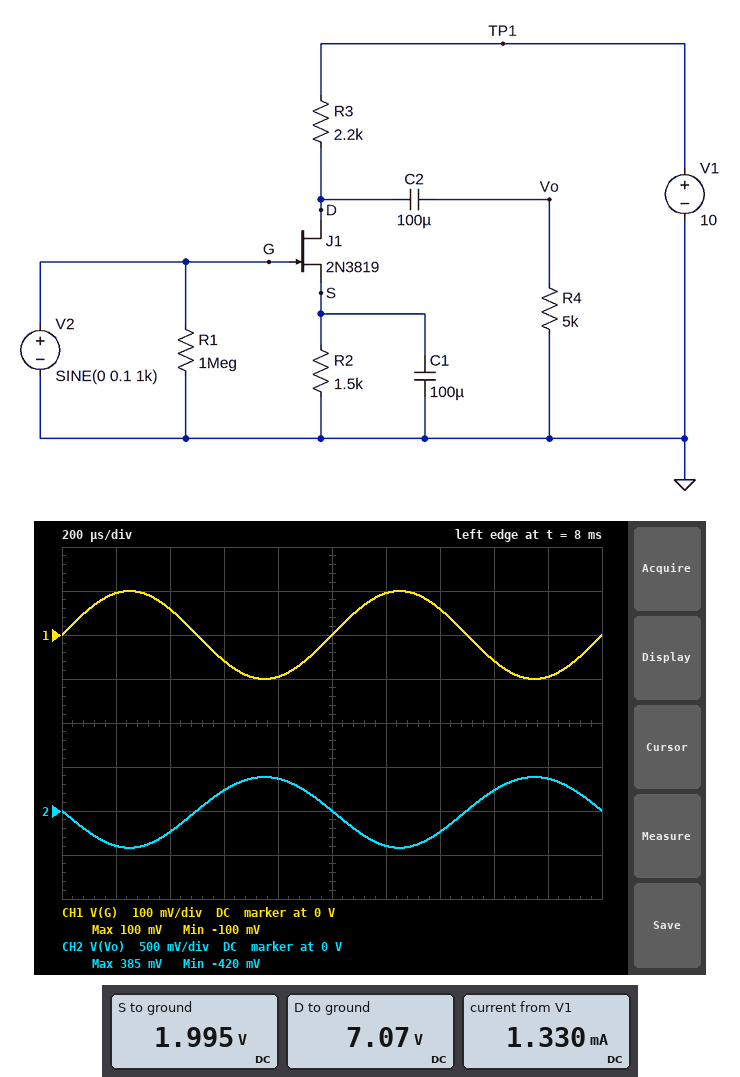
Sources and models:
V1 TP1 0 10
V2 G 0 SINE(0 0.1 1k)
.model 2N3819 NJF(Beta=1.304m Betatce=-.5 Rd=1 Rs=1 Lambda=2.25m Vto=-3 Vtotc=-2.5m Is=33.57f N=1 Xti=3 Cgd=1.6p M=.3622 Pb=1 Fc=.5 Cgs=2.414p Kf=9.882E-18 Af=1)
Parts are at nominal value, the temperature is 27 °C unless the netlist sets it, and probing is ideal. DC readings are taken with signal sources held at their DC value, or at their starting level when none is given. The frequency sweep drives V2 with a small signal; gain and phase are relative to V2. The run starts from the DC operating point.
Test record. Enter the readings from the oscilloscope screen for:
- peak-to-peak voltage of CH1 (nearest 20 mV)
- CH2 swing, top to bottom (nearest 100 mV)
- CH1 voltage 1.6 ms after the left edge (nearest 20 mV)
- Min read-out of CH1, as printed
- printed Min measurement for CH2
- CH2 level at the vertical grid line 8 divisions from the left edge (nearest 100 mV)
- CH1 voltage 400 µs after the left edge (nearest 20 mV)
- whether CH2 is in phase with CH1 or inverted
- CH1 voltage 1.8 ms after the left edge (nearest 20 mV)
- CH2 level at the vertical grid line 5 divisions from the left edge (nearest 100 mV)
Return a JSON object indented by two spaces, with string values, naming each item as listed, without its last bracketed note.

{
  "peak-to-peak voltage of CH1": "200 mV",
  "CH2 swing, top to bottom": "800 mV",
  "CH1 voltage 1.6 ms after the left edge": "-60 mV",
  "Min read-out of CH1, as printed": "-100 mV",
  "printed Min measurement for CH2": "-420 mV",
  "CH2 level at the vertical grid line 8 divisions from the left edge": "200 mV",
  "CH1 voltage 400 µs after the left edge": "60 mV",
  "whether CH2 is in phase with CH1 or inverted": "inverted",
  "CH1 voltage 1.8 ms after the left edge": "-100 mV",
  "CH2 level at the vertical grid line 5 divisions from the left edge": "0 V"
}
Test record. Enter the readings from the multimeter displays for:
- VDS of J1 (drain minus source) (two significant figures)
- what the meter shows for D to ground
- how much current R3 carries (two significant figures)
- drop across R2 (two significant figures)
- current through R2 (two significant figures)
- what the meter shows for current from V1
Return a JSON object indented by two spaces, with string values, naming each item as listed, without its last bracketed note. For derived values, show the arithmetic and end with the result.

{
  "VDS of J1 (drain minus source)": "7.07 V - 1.995 V = 5.1 V",
  "what the meter shows for D to ground": "7.07 V",
  "how much current R3 carries": "(10 V - 7.07 V) / 2.2 kΩ = 1.3 mA",
  "drop across R2": "1.995 V = 2.0 V",
  "current through R2": "(1.995 V) / 1.5 kΩ = 1.3 mA",
  "what the meter shows for current from V1": "1.330 mA"
}
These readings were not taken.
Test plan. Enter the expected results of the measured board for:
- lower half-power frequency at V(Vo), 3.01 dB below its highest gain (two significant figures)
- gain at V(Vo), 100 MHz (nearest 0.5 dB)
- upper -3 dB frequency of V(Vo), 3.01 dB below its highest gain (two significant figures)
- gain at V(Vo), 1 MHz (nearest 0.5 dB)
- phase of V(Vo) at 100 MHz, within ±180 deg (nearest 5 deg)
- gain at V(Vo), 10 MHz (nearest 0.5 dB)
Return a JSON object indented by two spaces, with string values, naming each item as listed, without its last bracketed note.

{
  "lower half-power frequency at V(Vo), 3.01 dB below its highest gain": "5.0 Hz",
  "gain at V(Vo), 100 MHz": "11.0 dB",
  "upper -3 dB frequency of V(Vo), 3.01 dB below its highest gain": "200 MHz",
  "gain at V(Vo), 1 MHz": "12.0 dB",
  "phase of V(Vo) at 100 MHz, within ±180 deg": "145 deg",
  "gain at V(Vo), 10 MHz": "12.0 dB"
}
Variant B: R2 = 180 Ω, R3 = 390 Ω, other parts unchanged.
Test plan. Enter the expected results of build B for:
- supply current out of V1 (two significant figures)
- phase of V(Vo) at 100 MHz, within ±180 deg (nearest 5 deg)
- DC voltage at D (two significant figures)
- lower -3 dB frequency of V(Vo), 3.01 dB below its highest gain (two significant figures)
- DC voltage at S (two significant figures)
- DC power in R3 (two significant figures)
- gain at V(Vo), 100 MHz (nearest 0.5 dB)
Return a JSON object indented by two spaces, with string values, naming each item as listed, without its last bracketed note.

{
  "supply current out of V1": "5.4 mA",
  "phase of V(Vo) at 100 MHz, within ±180 deg": "170 deg",
  "DC voltage at D": "7.9 V",
  "lower -3 dB frequency of V(Vo), 3.01 dB below its highest gain": "12 Hz",
  "DC voltage at S": "970 mV",
  "DC power in R3": "11 mW",
  "gain at V(Vo), 100 MHz": "5.5 dB"
}
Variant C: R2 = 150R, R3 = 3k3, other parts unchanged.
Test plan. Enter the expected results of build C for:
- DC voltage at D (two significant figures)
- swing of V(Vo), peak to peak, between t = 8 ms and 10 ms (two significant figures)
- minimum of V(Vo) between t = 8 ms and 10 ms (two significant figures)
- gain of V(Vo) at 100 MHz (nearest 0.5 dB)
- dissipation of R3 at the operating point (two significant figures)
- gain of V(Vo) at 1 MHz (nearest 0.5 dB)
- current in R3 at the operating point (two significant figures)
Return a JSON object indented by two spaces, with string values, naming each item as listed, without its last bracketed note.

{
  "DC voltage at D": "870 mV",
  "swing of V(Vo), peak to peak, between t = 8 ms and 10 ms": "39 mV",
  "minimum of V(Vo) between t = 8 ms and 10 ms": "-18 mV",
  "gain of V(Vo) at 100 MHz": "-13.0 dB",
  "dissipation of R3 at the operating point": "25 mW",
  "gain of V(Vo) at 1 MHz": "-14.5 dB",
  "current in R3 at the operating point": "2.8 mA"
}
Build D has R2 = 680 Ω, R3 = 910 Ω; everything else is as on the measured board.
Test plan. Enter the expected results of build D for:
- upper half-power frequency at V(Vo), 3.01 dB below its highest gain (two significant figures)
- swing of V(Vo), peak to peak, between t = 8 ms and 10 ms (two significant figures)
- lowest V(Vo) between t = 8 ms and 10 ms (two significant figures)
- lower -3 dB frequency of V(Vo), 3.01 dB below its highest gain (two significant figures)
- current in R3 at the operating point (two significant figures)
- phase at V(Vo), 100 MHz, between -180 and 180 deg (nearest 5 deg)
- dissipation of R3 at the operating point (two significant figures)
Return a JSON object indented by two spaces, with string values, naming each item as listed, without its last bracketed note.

{
  "upper half-power frequency at V(Vo), 3.01 dB below its highest gain": "450 MHz",
  "swing of V(Vo), peak to peak, between t = 8 ms and 10 ms": "550 mV",
  "lowest V(Vo) between t = 8 ms and 10 ms": "-280 mV",
  "lower -3 dB frequency of V(Vo), 3.01 dB below its highest gain": "7.3 Hz",
  "current in R3 at the operating point": "2.4 mA",
  "phase at V(Vo), 100 MHz, between -180 and 180 deg": "160 deg",
  "dissipation of R3 at the operating point": "5.3 mW"
}
